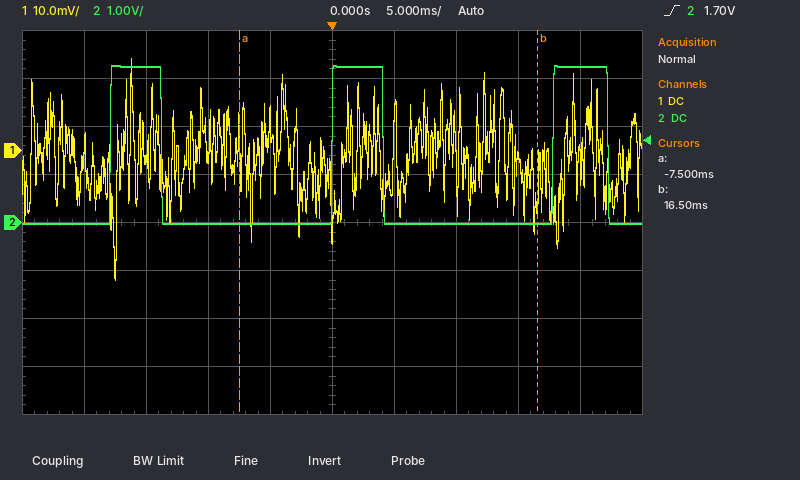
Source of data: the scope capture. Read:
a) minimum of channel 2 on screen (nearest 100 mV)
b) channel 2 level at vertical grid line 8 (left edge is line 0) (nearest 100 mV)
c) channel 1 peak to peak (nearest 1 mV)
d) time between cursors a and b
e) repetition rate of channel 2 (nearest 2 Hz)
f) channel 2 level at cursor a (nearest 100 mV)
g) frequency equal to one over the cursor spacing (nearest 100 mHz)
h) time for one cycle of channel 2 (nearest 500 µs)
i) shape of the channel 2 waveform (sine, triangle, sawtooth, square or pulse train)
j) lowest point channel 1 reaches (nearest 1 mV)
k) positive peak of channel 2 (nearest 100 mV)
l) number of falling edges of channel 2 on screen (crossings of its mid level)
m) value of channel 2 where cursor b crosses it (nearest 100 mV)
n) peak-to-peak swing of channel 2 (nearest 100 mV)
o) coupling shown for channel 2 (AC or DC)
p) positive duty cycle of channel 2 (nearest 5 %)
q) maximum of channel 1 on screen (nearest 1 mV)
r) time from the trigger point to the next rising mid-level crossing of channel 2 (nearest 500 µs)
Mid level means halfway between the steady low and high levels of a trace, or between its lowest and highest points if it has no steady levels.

0.0 V
0.0 V
46 mV
24.0 ms
56 Hz
0.0 V
41.7 Hz
18.0 ms
pulse train
-27 mV
3.3 V
3
0.0 V
3.3 V
DC
25 %
19 mV
18.0 ms
